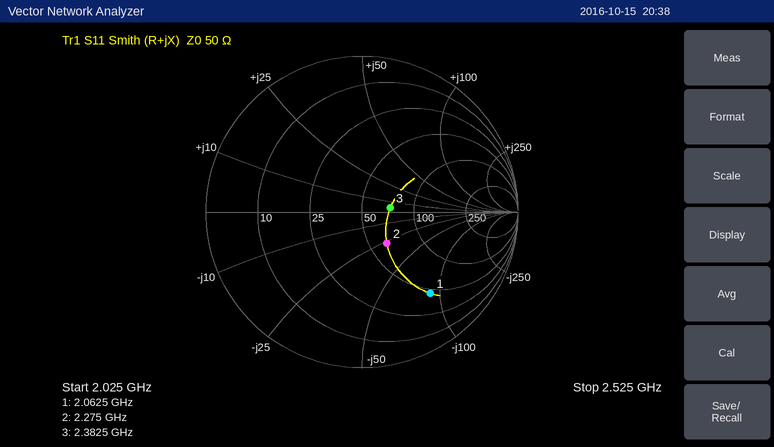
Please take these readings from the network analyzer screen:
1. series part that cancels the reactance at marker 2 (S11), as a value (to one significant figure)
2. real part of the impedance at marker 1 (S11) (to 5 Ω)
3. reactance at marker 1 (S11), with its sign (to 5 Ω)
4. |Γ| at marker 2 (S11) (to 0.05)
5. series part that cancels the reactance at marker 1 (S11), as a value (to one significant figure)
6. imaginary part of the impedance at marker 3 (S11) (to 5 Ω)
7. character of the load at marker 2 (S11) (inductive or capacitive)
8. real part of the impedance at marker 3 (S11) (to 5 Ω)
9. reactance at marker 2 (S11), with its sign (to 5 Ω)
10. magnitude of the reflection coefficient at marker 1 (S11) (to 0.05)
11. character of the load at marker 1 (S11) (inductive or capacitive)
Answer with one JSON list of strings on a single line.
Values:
["2 nH", "45 Ω", "-90 Ω", "0.25", "7 nH", "+5 Ω", "capacitive", "70 Ω", "-25 Ω", "0.70", "capacitive"]
